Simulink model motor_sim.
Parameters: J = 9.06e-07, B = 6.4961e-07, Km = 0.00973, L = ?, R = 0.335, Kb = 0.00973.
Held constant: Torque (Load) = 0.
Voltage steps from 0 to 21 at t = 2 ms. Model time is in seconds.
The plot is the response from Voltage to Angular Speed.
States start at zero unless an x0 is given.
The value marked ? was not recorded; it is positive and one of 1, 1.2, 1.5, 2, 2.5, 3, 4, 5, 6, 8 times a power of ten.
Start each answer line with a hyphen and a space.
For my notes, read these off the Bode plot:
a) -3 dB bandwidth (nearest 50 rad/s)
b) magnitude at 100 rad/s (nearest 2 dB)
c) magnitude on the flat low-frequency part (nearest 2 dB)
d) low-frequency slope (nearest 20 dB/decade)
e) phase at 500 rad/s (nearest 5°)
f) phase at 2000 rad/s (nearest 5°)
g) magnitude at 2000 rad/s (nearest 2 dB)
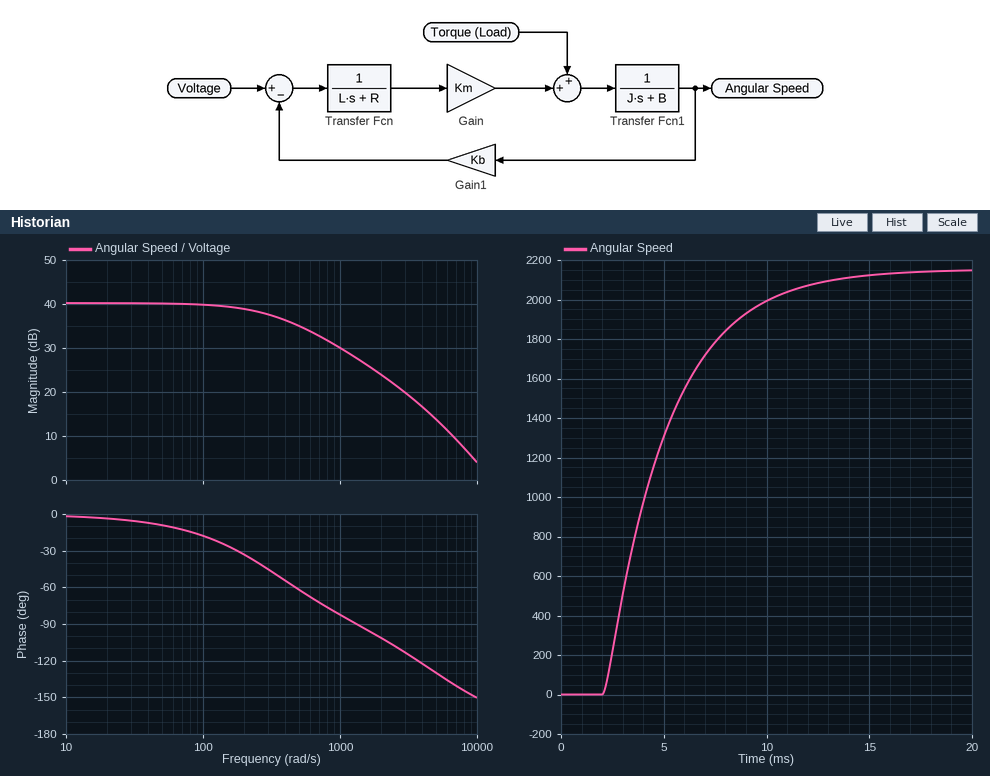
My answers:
- 350 rad/s
- 40 dB
- 40 dB
- 0 dB/decade
- -60°
- -100°
- 24 dB
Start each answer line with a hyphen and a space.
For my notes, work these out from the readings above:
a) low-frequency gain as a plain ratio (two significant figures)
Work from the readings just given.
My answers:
- 100
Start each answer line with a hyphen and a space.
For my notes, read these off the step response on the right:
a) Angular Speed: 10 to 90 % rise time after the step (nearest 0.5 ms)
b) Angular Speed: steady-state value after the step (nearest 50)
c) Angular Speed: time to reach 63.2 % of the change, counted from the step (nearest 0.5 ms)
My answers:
- 6.5 ms
- 2150
- 3.0 ms
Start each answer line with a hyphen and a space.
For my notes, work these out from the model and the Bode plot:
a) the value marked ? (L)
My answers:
- 6e-05
